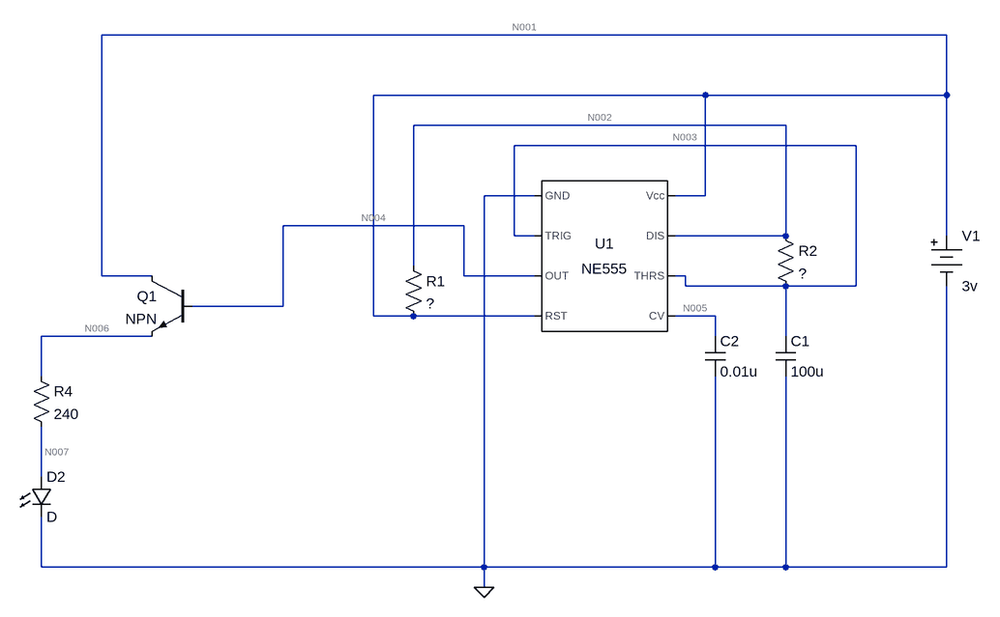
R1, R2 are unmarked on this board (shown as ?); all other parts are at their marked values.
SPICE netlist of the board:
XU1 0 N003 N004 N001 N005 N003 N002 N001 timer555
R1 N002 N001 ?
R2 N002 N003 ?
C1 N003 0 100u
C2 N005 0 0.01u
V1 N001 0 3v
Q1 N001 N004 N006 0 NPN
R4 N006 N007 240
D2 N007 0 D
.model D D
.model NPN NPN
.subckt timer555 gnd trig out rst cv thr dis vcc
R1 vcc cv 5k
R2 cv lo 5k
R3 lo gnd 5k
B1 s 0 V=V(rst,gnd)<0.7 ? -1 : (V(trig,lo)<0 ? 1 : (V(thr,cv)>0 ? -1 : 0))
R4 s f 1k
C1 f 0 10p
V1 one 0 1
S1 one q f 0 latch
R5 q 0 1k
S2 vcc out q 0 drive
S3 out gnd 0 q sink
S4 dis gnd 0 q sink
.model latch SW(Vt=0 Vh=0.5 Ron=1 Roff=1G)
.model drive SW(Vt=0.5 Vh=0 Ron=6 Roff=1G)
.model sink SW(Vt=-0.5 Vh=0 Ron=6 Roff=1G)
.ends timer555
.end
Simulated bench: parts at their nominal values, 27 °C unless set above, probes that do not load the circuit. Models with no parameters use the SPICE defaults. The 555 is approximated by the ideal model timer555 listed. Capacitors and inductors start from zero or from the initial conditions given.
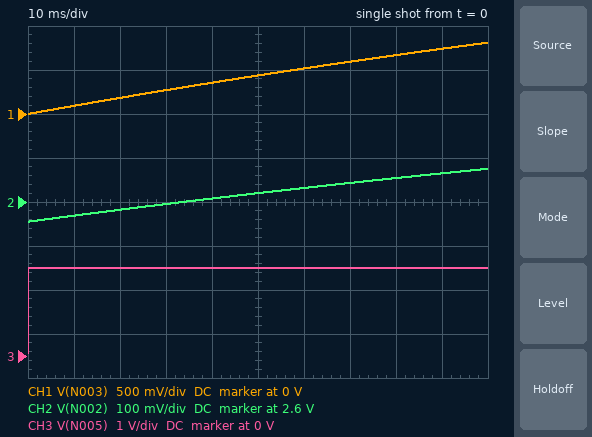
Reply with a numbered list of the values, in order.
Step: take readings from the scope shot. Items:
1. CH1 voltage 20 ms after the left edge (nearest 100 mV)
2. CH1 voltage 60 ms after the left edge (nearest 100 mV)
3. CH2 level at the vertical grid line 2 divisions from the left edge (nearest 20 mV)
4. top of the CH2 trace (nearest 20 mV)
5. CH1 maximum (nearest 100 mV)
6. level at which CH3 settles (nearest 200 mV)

1. 200 mV
2. 500 mV
3. 2.58 V
4. 2.68 V
5. 800 mV
6. 2.0 V
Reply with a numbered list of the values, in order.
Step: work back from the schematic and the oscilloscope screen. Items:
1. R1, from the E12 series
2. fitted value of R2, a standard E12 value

1. 470 Ω
2. 2.7 kΩ
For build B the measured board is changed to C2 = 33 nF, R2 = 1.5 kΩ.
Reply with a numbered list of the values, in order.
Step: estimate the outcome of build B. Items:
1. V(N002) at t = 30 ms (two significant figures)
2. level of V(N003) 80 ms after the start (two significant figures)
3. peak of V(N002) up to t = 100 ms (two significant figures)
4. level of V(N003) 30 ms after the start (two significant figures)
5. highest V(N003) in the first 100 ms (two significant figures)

1. 2.4 V
2. 1.0 V
3. 2.6 V
4. 420 mV
5. 1.2 V
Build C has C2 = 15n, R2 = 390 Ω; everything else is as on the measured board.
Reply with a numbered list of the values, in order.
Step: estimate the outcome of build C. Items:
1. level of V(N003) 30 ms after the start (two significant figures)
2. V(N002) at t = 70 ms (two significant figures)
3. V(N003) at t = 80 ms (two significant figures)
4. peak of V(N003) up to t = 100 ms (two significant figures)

1. 880 mV
2. 2.3 V
3. 1.8 V
4. 2.0 V
